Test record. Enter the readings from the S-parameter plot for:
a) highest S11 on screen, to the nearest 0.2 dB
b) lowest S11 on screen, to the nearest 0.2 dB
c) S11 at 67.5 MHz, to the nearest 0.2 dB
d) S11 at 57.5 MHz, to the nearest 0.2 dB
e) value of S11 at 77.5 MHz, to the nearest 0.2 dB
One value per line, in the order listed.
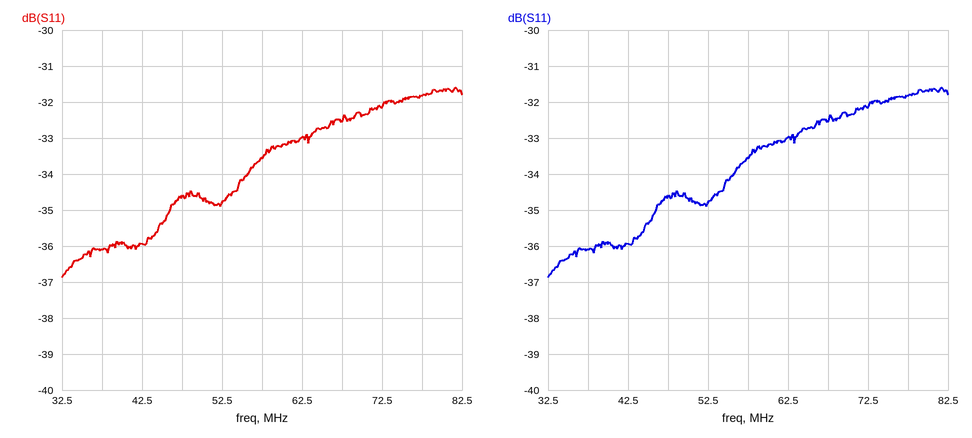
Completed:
-31.6 dB
-36.8 dB
-32.6 dB
-33.6 dB
-31.8 dB
